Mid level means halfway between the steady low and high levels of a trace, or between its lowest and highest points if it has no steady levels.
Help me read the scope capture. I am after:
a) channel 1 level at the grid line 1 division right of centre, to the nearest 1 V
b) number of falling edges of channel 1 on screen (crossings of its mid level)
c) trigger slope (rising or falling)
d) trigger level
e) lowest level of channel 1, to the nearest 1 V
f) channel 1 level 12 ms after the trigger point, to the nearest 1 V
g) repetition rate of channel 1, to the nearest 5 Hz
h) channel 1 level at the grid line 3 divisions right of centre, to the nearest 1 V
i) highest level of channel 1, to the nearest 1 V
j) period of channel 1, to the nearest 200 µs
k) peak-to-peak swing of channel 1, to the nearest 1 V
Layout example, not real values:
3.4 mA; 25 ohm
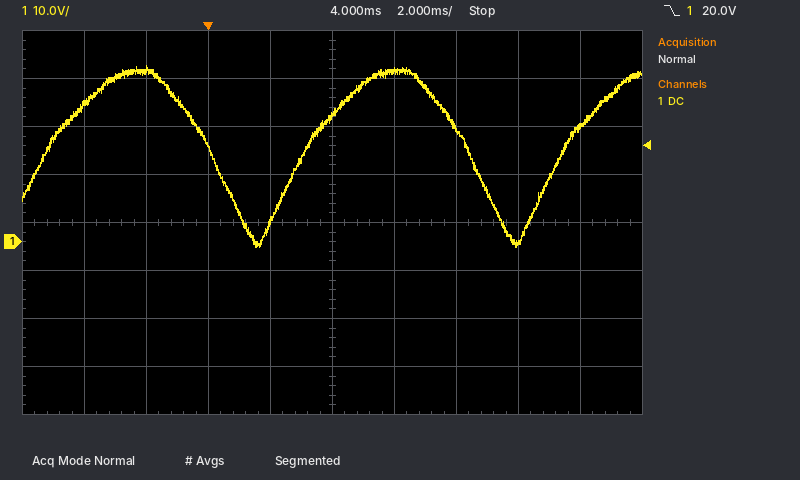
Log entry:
36 V; 2; falling; 20.0 V; -1 V; 24 V; 120 Hz; 0 V; 37 V; 8.4 ms; 38 V
